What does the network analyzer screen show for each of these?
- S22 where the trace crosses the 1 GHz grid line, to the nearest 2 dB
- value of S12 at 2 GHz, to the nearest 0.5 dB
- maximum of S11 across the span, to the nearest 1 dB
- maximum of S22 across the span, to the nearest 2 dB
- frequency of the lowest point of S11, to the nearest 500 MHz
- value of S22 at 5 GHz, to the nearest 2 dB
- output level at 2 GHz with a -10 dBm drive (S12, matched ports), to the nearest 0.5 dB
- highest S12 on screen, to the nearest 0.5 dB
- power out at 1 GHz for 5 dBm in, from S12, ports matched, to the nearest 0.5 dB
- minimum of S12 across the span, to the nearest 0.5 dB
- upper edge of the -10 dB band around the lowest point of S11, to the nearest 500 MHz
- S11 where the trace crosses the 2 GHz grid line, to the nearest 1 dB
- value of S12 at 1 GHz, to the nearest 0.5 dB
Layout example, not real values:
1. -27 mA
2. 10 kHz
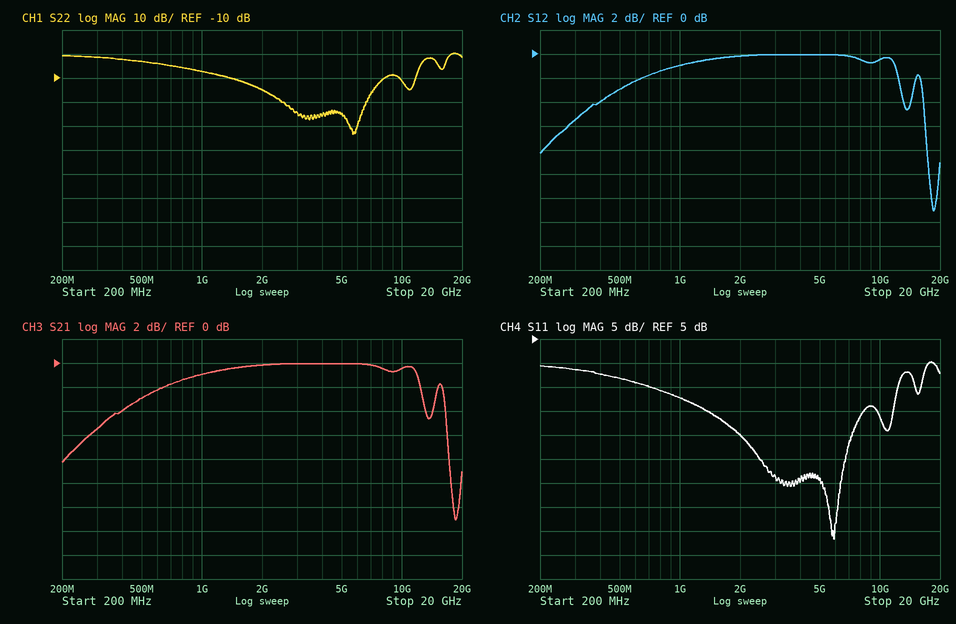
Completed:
1. -8 dB
2. 0.0 dB
3. 0 dB
4. 0 dB
5. 6.0 GHz
6. -24 dB
7. -10.0 dBm
8. 0.0 dB
9. 4.0 dBm
10. -13.0 dB
11. 8.5 GHz
12. -15 dB
13. -1.0 dB
